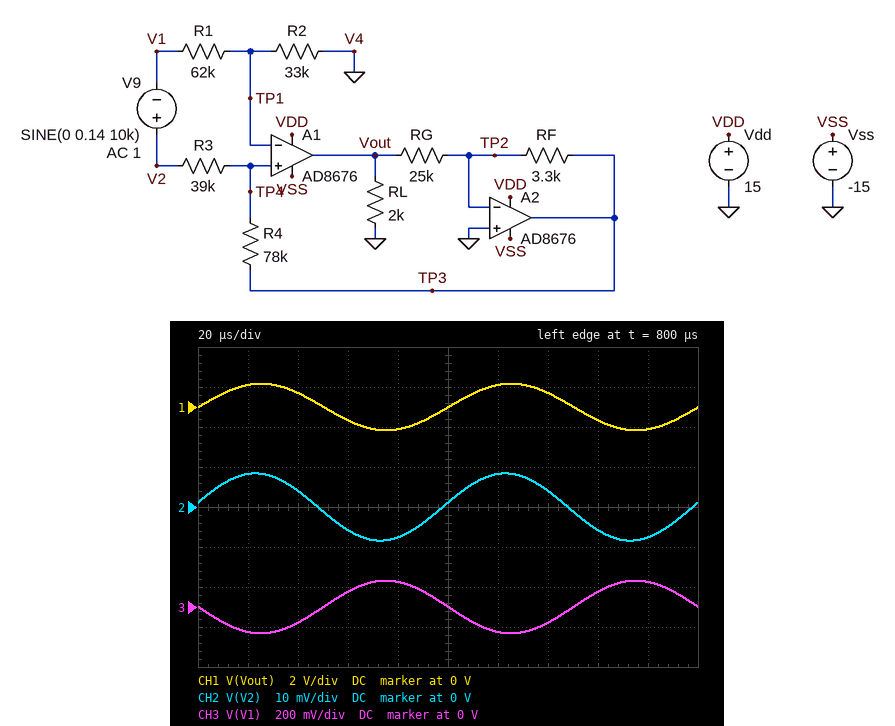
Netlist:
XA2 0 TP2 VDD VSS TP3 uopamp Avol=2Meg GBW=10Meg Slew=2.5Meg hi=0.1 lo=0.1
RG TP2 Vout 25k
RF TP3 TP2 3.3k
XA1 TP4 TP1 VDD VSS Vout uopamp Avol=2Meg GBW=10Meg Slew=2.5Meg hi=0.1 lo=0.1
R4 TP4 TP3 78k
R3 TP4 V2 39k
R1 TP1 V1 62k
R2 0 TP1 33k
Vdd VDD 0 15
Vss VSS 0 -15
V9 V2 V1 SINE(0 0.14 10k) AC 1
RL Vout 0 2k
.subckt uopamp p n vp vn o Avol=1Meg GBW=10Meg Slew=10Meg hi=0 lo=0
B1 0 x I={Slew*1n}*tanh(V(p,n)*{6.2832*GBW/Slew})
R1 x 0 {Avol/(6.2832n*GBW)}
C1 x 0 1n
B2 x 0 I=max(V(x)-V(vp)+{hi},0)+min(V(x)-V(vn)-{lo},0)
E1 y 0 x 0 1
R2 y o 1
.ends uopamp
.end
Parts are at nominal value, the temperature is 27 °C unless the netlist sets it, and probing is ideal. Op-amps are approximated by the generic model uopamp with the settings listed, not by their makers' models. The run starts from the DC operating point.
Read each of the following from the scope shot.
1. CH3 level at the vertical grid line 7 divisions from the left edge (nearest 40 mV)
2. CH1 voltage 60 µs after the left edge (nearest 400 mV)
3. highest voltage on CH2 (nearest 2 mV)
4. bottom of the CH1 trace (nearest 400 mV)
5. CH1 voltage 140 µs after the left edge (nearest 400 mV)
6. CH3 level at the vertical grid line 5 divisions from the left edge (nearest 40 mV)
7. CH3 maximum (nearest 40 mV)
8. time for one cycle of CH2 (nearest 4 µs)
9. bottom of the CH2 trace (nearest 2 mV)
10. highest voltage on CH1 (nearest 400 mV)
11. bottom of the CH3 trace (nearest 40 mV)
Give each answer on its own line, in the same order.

-80 mV
-800 mV
8 mV
-1.2 V
800 mV
0 V
120 mV
100 µs
-8 mV
1.2 V
-120 mV
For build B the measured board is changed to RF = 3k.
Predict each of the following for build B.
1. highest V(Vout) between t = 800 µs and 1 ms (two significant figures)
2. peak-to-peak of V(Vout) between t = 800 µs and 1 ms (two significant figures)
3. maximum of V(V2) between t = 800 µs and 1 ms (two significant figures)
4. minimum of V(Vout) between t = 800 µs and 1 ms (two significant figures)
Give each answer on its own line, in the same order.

1.3 V
2.6 V
8.4 mV
-1.3 V
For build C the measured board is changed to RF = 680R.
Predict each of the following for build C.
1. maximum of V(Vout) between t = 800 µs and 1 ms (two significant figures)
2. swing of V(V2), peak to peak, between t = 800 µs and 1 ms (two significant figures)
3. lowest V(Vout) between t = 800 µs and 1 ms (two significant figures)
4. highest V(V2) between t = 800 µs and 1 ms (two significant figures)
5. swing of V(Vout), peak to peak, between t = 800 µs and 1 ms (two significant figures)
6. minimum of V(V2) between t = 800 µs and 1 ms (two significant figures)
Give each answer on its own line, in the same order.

5.6 V
20 mV
-5.6 V
10 mV
11 V
-10 mV
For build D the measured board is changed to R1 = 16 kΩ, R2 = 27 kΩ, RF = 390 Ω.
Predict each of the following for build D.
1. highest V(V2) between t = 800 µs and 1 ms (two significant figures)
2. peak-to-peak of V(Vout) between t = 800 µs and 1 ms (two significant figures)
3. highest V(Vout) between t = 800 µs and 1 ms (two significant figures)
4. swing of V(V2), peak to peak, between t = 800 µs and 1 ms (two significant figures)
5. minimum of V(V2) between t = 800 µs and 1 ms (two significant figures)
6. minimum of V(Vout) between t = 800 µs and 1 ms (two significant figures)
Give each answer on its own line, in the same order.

40 mV
30 V
15 V
80 mV
-40 mV
-15 V
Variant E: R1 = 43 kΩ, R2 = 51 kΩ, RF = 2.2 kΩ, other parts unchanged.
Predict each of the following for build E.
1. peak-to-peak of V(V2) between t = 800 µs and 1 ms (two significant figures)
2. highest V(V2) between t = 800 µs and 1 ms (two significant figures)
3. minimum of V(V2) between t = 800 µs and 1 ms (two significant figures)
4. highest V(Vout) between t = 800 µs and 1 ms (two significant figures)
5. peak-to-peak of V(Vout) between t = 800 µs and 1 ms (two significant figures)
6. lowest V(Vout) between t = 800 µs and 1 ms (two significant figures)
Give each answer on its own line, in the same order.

41 mV
21 mV
-21 mV
2.5 V
5.0 V
-2.5 V
